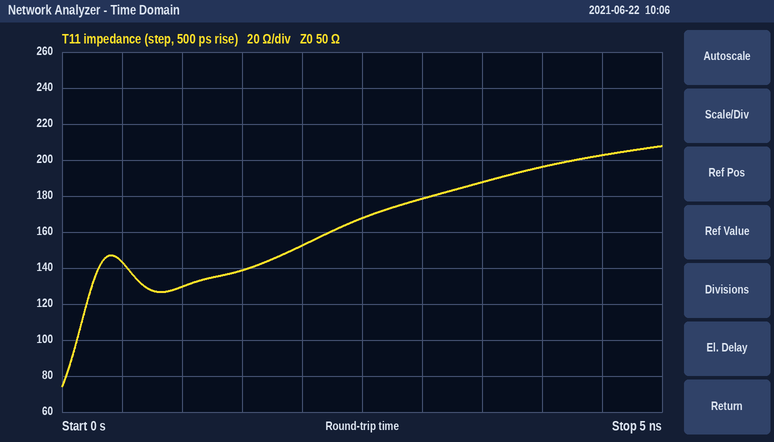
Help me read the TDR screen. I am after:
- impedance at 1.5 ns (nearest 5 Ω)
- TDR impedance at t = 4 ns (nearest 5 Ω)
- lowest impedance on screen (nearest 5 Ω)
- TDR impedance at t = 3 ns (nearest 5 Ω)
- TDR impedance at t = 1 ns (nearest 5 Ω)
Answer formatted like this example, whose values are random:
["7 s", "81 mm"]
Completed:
["140 Ω", "195 Ω", "75 Ω", "180 Ω", "130 Ω"]
